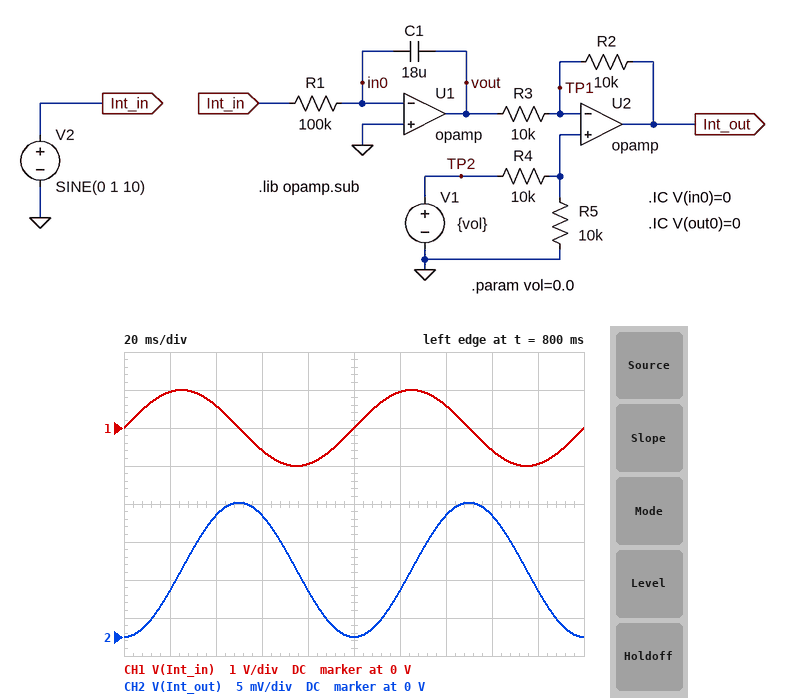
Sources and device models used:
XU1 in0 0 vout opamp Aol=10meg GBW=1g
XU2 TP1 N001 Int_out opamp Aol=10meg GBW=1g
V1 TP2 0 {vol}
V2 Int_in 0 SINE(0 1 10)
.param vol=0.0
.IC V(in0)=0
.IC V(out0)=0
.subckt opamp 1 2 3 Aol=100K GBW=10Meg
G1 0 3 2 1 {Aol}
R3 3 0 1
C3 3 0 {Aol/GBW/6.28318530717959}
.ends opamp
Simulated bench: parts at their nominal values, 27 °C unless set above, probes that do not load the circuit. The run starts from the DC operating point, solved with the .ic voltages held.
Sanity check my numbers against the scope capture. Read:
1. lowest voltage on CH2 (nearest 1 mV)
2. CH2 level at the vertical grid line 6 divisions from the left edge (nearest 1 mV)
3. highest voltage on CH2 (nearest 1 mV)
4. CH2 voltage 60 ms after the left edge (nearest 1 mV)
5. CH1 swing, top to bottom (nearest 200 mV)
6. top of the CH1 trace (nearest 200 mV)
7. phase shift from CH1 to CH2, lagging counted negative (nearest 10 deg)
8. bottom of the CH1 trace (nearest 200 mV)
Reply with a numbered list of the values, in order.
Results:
1. 0 V
2. 6 mV
3. 18 mV
4. 16 mV
5. 2.0 V
6. 1.0 V
7. -90 deg
8. -1.0 V
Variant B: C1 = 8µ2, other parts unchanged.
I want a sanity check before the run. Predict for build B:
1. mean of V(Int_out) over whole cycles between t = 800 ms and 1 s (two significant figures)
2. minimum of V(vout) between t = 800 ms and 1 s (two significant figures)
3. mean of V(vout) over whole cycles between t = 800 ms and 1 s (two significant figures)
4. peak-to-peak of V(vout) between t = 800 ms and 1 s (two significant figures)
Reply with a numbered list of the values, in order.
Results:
1. 19 mV
2. -39 mV
3. -19 mV
4. 39 mV
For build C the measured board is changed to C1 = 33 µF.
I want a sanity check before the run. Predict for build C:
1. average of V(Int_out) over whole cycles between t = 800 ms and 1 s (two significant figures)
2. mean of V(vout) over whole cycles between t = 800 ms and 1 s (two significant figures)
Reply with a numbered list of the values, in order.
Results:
1. 4.8 mV
2. -4.8 mV
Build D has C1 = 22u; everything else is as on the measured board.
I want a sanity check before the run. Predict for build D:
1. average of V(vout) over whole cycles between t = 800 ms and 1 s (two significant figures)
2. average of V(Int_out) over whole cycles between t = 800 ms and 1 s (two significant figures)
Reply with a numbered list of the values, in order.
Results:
1. -7.2 mV
2. 7.2 mV
